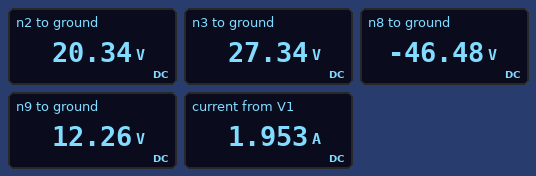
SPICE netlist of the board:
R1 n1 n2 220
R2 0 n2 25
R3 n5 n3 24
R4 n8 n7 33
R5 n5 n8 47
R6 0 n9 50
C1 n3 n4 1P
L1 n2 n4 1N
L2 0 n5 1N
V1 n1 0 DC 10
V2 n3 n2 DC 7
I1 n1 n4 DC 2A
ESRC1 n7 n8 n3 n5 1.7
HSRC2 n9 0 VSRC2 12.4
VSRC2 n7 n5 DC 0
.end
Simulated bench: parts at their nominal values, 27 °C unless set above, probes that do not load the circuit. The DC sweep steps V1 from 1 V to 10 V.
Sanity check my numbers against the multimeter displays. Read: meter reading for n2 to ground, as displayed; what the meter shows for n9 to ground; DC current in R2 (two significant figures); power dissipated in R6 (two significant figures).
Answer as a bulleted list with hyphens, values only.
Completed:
- 20.34 V
- 12.26 V
- 810 mA
- 3.0 W
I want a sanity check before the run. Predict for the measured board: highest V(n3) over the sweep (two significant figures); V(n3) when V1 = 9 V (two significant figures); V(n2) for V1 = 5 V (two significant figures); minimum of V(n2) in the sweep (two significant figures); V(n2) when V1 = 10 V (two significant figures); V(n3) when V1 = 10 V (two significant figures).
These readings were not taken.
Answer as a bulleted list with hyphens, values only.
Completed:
- 27 V
- 27 V
- 20 V
- 20 V
- 20 V
- 27 V
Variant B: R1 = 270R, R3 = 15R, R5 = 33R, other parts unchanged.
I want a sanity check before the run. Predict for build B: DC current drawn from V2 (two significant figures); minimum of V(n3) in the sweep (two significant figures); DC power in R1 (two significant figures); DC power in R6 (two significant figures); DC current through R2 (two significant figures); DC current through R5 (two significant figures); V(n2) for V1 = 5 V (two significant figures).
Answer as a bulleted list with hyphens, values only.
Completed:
- 1.4 A
- 21 V
- 66 mW
- 3.7 W
- 570 mA
- 1.1 A
- 14 V
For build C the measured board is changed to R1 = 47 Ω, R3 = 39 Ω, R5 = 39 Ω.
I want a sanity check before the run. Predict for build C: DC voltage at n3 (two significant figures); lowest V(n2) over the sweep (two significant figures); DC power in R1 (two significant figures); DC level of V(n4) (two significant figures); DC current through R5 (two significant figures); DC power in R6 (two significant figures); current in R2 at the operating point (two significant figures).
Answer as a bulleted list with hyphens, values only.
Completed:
- 30 V
- 21 V
- 3.8 W
- 23 V
- 1.3 A
- 5.4 W
- 940 mA
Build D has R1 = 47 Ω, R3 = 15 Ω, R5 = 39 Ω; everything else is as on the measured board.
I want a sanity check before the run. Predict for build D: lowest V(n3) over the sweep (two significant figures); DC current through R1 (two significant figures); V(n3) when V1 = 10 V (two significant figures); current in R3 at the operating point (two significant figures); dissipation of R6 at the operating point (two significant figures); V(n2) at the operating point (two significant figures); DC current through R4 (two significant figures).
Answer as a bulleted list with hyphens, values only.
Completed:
- 19 V
- 78 mA
- 21 V
- 1.4 A
- 2.5 W
- 14 V
- 1.1 A
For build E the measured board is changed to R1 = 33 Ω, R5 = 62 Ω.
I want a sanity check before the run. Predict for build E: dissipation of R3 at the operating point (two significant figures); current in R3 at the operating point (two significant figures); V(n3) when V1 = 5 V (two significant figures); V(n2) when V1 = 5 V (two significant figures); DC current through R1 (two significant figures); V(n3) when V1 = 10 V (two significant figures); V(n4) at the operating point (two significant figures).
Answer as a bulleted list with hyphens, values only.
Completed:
- 26 W
- 1.0 A
- 24 V
- 17 V
- 240 mA
- 25 V
- 18 V
